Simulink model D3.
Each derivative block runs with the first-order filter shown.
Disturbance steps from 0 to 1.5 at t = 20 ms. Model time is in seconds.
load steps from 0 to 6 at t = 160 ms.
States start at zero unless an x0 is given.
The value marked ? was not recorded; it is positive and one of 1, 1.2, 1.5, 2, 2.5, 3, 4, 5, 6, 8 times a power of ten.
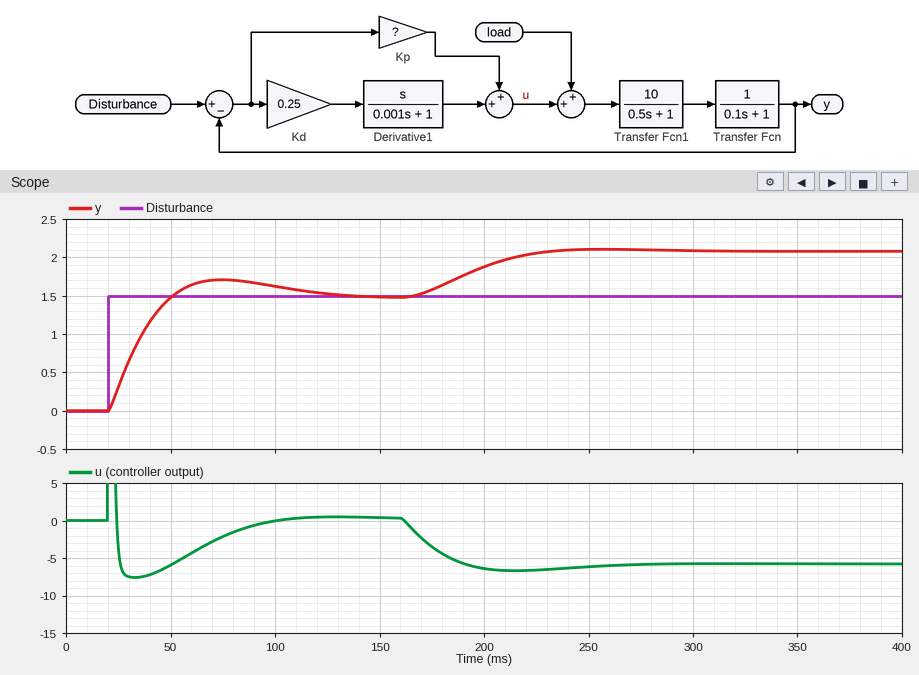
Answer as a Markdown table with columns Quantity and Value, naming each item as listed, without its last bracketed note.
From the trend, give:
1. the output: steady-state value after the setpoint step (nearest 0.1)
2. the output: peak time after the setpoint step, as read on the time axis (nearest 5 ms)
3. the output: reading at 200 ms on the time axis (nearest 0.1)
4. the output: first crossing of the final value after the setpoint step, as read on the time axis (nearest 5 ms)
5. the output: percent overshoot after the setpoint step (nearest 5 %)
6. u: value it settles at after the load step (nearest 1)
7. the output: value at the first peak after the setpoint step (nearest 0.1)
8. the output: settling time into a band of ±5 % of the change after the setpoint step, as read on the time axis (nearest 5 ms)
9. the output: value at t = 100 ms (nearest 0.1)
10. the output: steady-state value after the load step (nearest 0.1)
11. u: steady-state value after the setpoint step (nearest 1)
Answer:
| Quantity | Value |
|---|---|
| the output: steady-state value after the setpoint step | 1.5 |
| the output: peak time after the setpoint step, as read on the time axis | 75 ms |
| the output: reading at 200 ms on the time axis | 1.9 |
| the output: first crossing of the final value after the setpoint step, as read on the time axis | 50 ms |
| the output: percent overshoot after the setpoint step | 15 % |
| u: value it settles at after the load step | -6 |
| the output: value at the first peak after the setpoint step | 1.7 |
| the output: settling time into a band of ±5 % of the change after the setpoint step, as read on the time axis | 115 ms |
| the output: value at t = 100 ms | 1.6 |
| the output: steady-state value after the load step | 2.1 |
| u: steady-state value after the setpoint step | 0 |
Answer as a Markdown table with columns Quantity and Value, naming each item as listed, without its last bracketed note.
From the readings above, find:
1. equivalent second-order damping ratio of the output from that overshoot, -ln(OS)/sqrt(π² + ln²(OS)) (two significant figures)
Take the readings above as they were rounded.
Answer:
| Quantity | Value |
|---|---|
| equivalent second-order damping ratio of the output from that overshoot, -ln(OS)/sqrt(π² + ln²(OS)) | 0.52 |
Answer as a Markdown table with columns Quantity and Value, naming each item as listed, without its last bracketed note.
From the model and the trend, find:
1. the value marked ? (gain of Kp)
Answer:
| Quantity | Value |
|---|---|
| the value marked ? | 10 |
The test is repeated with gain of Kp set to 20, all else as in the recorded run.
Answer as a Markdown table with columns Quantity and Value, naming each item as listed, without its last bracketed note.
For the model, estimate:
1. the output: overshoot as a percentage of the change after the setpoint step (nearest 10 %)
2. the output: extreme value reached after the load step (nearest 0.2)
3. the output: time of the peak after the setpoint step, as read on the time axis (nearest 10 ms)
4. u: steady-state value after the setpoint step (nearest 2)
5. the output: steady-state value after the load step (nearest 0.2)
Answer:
| Quantity | Value |
|---|---|
| the output: overshoot as a percentage of the change after the setpoint step | 30 % |
| the output: extreme value reached after the load step | 1.8 |
| the output: time of the peak after the setpoint step, as read on the time axis | 60 ms |
| u: steady-state value after the setpoint step | 0 |
| the output: steady-state value after the load step | 1.8 |
